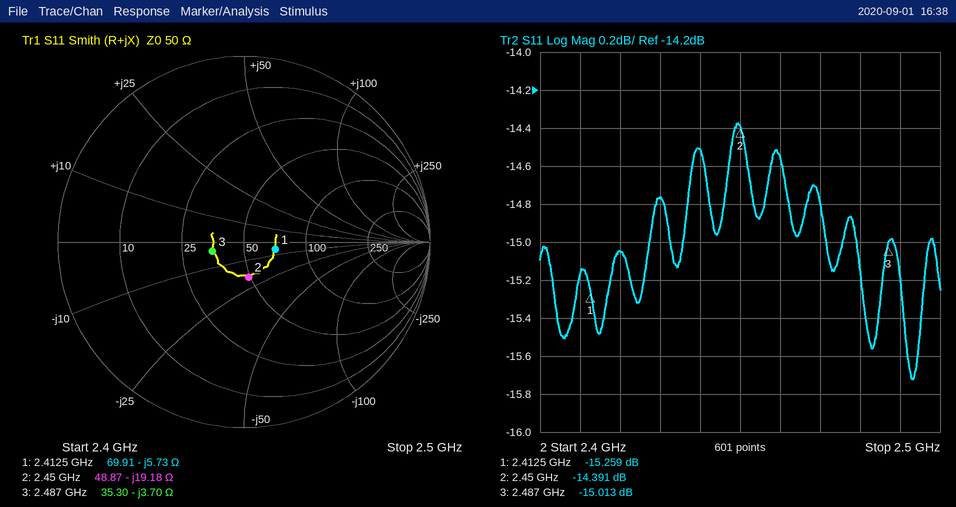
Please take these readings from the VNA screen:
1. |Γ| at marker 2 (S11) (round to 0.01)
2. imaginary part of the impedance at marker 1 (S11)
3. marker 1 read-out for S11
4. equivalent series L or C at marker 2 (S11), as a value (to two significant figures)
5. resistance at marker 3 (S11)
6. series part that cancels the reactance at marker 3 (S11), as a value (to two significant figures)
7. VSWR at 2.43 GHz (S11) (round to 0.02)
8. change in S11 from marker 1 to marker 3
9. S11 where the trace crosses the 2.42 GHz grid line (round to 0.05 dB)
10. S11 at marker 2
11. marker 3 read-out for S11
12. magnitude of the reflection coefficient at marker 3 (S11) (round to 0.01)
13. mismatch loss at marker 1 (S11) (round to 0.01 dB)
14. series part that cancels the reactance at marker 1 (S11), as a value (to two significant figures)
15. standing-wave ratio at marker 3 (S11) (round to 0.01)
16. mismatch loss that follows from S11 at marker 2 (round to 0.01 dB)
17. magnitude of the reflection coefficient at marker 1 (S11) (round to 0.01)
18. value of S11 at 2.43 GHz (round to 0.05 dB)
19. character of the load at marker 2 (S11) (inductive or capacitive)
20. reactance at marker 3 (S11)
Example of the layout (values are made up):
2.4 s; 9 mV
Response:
0.19; -5.73 Ω; -15.259 dB; 3.4 pF; 35.30 Ω; 240 pH; 1.44; 0.246 dB; -15.05 dB; -14.391 dB; -15.013 dB; 0.18; 0.13 dB; 380 pH; 1.43; 0.16 dB; 0.17; -14.75 dB; capacitive; -3.70 Ω
